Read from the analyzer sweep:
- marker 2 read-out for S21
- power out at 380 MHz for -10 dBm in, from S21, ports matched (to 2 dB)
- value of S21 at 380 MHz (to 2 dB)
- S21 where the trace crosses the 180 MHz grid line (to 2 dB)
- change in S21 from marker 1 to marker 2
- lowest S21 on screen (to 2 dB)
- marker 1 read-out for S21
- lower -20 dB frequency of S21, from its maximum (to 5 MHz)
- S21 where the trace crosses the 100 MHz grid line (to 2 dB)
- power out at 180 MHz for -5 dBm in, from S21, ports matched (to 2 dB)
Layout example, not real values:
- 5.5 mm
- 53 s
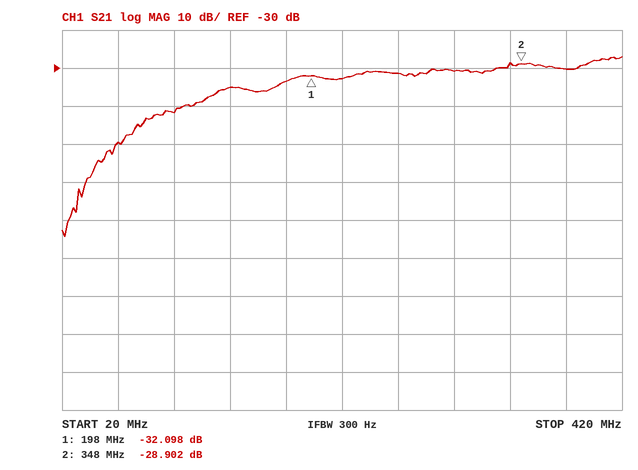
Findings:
- -28.902 dB
- -40 dBm
- -30 dB
- -34 dB
- 3.196 dB
- -74 dB
- -32.098 dB
- 70 MHz
- -42 dB
- -38 dBm
